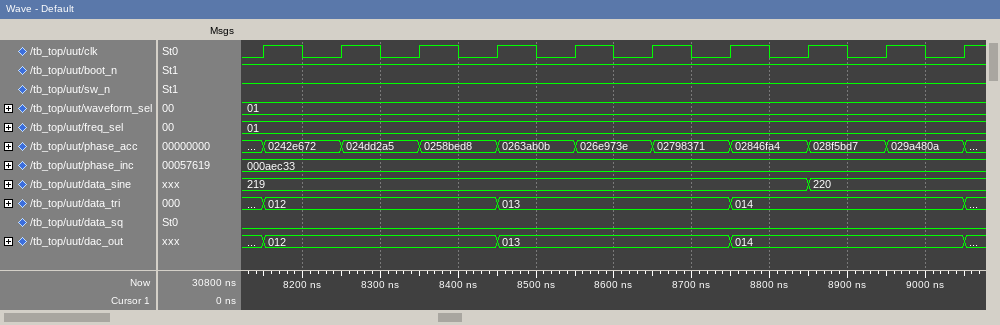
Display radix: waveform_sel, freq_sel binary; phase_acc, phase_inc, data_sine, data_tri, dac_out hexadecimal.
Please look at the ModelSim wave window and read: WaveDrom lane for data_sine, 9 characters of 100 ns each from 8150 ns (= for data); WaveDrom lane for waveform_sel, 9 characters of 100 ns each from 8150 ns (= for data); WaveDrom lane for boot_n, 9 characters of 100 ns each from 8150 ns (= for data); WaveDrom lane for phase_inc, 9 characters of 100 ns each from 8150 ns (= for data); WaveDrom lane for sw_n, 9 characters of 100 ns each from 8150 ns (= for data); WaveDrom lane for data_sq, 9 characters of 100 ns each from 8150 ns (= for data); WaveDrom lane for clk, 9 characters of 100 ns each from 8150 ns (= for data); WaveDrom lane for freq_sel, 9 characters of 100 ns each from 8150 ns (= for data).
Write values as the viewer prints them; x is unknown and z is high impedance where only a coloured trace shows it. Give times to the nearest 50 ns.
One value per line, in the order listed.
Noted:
{name: 'data_sine', wave: '=......=.', data: '219 220'}
{name: 'waveform_sel', wave: '=........', data: '01'}
{name: 'boot_n', wave: '1........'}
{name: 'phase_inc', wave: '=........', data: '000aec33'}
{name: 'sw_n', wave: '1........'}
{name: 'data_sq', wave: '0........'}
{name: 'clk', wave: 'p........'}
{name: 'freq_sel', wave: '=........', data: '01'}
